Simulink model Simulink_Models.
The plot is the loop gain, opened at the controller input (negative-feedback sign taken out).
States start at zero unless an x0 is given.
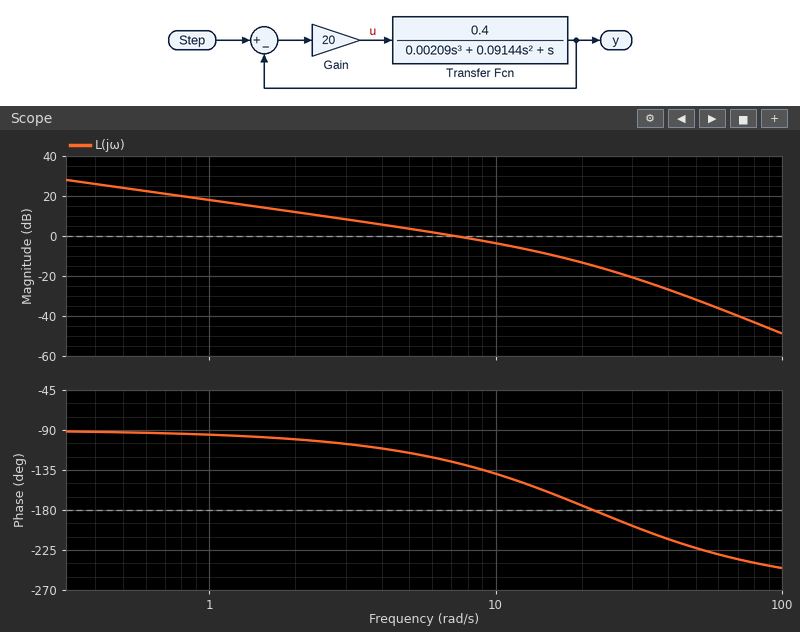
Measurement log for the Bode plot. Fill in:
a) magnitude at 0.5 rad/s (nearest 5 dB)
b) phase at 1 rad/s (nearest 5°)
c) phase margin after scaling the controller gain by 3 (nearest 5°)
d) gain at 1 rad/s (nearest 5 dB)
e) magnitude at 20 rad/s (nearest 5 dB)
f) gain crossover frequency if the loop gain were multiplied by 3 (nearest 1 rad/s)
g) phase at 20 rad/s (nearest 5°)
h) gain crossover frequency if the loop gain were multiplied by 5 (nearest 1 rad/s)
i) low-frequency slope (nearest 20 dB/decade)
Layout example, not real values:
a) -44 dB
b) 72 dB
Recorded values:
a) 25 dB
b) -95°
c) 20°
d) 20 dB
e) -15 dB
f) 16 rad/s
g) -175°
h) 21 rad/s
i) -20 dB/decade
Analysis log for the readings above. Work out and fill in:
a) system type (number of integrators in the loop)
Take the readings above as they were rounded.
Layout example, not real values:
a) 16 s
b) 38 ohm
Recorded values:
a) 1
